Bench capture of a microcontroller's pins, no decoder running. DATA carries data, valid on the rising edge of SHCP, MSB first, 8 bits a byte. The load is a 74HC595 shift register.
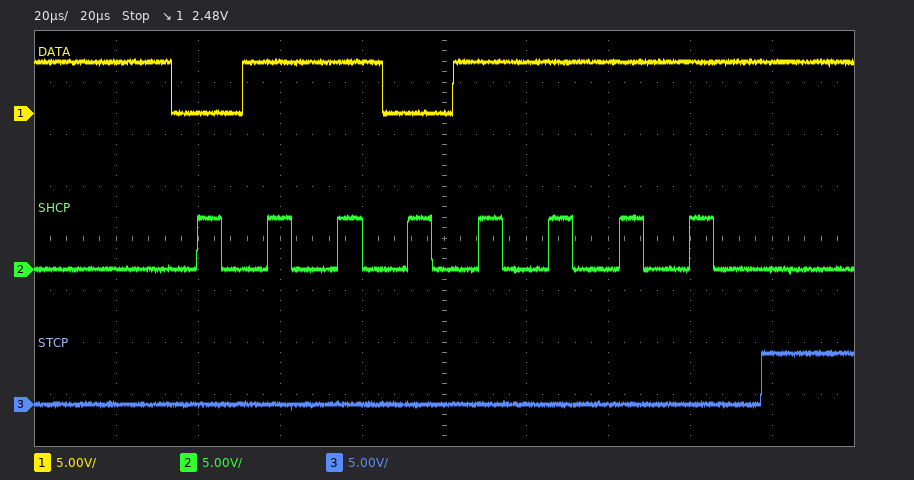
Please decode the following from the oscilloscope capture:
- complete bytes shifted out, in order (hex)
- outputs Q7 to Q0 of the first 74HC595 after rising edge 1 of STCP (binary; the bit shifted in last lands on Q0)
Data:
0x6F
01101111
